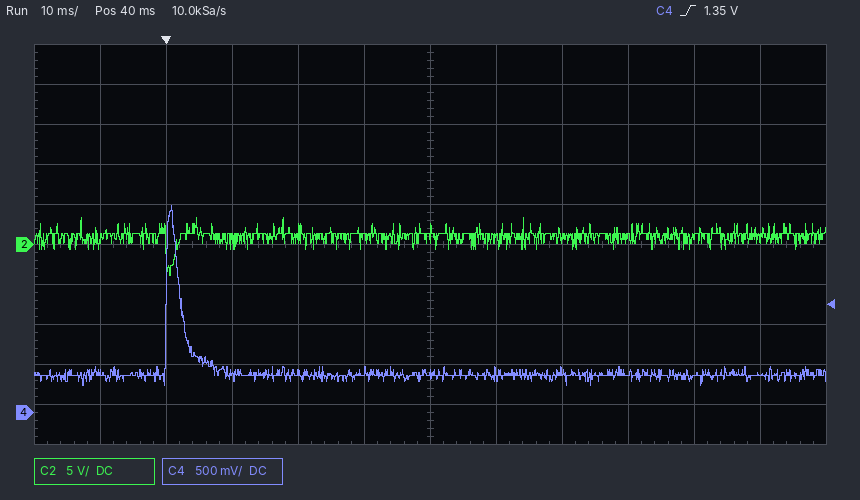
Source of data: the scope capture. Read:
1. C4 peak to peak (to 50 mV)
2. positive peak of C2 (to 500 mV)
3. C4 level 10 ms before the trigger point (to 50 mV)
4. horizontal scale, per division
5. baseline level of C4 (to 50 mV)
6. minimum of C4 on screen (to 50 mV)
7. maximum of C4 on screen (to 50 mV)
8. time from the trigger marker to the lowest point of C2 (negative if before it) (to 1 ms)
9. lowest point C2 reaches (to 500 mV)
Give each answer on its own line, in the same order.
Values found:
2.25 V
3.5 V
500 mV
10 ms
450 mV
350 mV
2.60 V
+1 ms
-4.0 V
